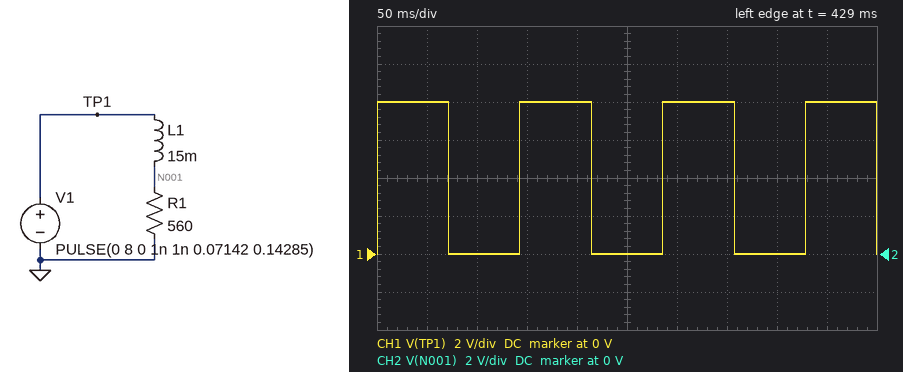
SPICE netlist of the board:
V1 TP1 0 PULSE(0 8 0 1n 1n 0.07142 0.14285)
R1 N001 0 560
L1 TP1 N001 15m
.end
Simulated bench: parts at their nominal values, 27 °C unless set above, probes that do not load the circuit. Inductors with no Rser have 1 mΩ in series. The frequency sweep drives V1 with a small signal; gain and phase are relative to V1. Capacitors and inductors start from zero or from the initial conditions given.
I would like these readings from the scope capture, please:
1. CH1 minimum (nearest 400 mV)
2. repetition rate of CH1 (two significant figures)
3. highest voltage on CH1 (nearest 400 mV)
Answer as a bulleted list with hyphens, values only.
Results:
- 0 V
- 7.0 Hz
- 8.0 V
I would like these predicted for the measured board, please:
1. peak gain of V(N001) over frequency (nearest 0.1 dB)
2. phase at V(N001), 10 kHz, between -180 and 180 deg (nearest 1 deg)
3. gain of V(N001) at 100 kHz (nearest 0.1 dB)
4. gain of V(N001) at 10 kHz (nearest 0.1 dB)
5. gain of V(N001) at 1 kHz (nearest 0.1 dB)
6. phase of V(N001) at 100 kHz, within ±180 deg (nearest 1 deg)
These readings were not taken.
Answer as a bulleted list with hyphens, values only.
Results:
- 0 dB
- -59 deg
- -24.5 dB
- -5.8 dB
- -0.1 dB
- -87 deg
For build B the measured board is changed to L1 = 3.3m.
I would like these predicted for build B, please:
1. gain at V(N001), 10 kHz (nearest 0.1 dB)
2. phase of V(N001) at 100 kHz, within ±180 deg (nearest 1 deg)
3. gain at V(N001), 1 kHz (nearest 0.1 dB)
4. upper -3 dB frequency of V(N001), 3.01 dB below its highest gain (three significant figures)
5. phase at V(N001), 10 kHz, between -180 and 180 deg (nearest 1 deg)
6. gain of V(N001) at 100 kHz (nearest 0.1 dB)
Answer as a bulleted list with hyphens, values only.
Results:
- -0.6 dB
- -75 deg
- 0 dB
- 27.0 kHz
- -20 deg
- -11.7 dB
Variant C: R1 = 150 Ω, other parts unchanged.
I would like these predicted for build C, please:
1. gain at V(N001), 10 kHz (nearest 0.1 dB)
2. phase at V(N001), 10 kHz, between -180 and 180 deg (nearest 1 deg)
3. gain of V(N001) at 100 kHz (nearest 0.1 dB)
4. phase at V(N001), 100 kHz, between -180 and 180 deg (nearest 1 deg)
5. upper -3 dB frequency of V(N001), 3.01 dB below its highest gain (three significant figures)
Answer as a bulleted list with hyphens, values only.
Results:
- -16.1 dB
- -81 deg
- -36.0 dB
- -89 deg
- 1.59 kHz
